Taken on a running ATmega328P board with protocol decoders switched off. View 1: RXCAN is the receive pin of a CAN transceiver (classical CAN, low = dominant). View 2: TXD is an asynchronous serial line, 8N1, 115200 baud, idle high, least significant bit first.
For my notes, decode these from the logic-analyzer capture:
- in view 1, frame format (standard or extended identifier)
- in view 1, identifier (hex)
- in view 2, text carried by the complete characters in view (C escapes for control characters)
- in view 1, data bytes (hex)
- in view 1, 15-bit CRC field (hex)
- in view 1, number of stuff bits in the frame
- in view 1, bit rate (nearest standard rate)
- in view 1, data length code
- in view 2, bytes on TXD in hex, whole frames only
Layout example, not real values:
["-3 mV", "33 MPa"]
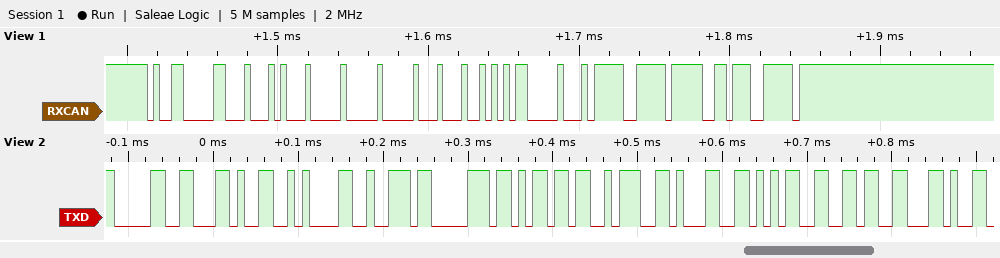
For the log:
["standard", "0x4C1", "\"0,\\nrpm:156,\"", "A2 00 00 44 AB 00 BE FF", "0x6DCF", "8", "250 kbit/s", "8", "30 2C 0A 72 70 6D 3A 31 35 36 2C"]
